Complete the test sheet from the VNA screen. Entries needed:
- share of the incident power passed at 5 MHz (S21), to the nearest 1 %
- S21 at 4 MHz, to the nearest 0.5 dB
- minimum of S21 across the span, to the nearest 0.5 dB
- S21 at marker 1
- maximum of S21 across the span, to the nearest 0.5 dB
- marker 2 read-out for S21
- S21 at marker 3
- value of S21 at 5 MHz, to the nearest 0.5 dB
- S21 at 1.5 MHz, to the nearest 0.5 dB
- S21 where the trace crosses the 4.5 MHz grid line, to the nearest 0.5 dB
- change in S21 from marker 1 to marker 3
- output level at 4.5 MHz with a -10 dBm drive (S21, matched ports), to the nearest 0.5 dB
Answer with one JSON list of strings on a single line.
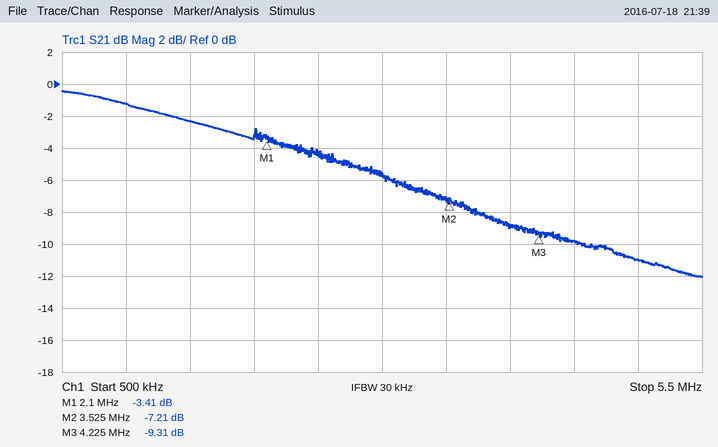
["8 %", "-9.0 dB", "-12.0 dB", "-3.41 dB", "-0.5 dB", "-7.21 dB", "-9.31 dB", "-11.0 dB", "-2.5 dB", "-10.0 dB", "-5.90 dB", "-20.0 dBm"]
